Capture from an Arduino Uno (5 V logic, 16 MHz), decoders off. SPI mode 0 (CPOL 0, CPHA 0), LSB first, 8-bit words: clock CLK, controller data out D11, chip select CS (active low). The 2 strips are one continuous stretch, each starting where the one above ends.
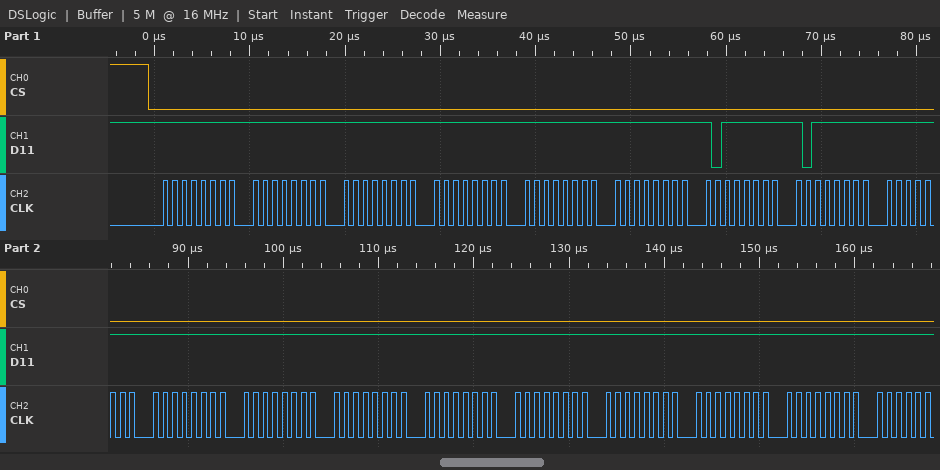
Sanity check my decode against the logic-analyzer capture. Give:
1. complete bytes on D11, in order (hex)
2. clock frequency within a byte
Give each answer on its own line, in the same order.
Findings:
FF FF FF FF FF FF FD FD FF FF FF FF FF FF FF FF FF
1 MHz
